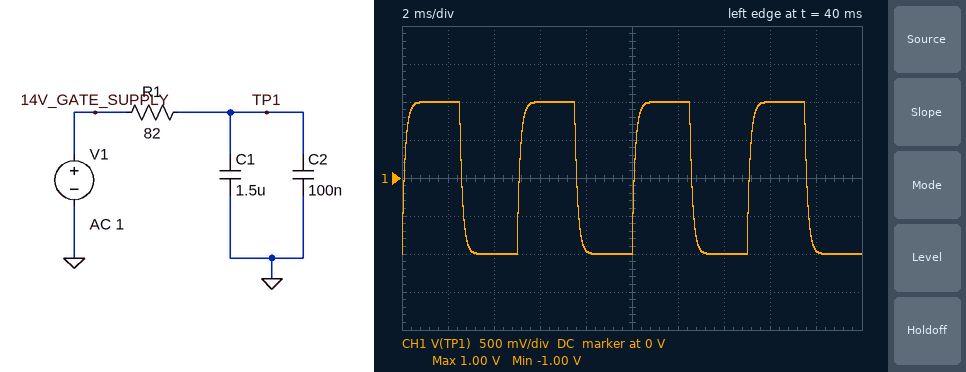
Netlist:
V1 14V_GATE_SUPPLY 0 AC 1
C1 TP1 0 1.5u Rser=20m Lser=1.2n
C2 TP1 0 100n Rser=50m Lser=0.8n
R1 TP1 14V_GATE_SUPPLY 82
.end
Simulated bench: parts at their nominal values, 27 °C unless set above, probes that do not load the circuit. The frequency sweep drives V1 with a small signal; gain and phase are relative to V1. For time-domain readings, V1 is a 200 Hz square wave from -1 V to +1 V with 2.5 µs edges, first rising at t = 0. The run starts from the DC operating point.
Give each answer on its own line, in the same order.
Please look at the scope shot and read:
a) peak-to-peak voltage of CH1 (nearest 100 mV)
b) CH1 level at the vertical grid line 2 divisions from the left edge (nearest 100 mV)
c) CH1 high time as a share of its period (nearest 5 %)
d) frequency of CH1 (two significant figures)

2.0 V
-1.0 V
50 %
200 Hz
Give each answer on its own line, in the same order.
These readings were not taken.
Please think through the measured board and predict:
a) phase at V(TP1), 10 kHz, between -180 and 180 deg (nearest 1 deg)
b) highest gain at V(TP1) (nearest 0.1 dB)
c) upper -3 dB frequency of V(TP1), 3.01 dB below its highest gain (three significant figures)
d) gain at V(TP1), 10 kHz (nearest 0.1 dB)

-83 deg
0 dB
1.21 kHz
-18.4 dB
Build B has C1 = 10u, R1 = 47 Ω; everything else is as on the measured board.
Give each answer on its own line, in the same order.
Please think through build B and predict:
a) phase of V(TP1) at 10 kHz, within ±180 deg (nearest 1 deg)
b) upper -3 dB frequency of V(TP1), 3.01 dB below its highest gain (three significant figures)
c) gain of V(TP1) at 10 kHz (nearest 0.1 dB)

-87 deg
335 Hz
-29.5 dB
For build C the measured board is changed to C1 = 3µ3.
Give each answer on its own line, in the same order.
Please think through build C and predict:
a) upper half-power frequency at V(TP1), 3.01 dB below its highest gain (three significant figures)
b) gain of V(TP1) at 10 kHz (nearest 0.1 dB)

571 Hz
-24.9 dB
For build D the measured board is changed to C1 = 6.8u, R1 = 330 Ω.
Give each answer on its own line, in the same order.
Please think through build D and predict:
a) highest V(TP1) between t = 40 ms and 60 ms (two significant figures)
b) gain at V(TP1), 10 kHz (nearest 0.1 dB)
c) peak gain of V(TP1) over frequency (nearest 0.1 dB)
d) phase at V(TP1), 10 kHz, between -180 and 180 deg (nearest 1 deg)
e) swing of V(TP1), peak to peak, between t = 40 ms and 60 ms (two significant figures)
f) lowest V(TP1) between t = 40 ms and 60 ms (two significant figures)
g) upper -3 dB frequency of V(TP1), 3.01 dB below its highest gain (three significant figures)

500 mV
-43.1 dB
0 dB
-89 deg
1.0 V
-500 mV
69.9 Hz
